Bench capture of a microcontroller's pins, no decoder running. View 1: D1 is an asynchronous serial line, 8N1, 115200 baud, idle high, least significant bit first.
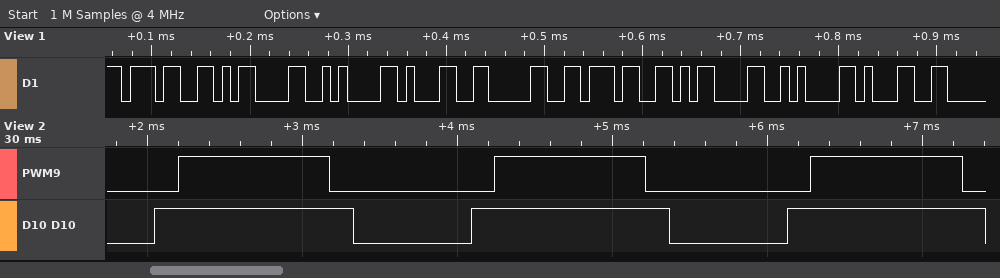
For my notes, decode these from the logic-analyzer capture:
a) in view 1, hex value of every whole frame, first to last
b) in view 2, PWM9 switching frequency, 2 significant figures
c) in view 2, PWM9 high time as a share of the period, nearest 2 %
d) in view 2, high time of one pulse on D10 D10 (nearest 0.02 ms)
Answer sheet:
0x37 0x0D 0x0A 0x31 0x30 0x37 0x0D 0x0A 0x31
490 Hz
48 %
1.28 ms
